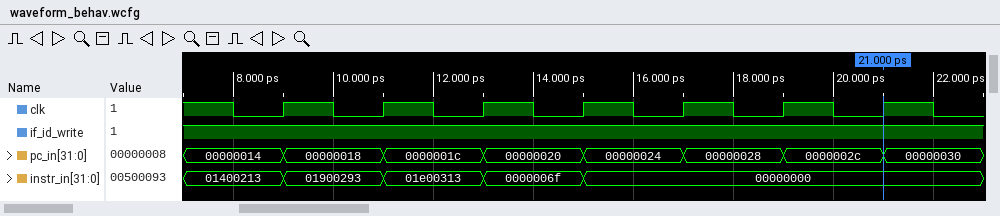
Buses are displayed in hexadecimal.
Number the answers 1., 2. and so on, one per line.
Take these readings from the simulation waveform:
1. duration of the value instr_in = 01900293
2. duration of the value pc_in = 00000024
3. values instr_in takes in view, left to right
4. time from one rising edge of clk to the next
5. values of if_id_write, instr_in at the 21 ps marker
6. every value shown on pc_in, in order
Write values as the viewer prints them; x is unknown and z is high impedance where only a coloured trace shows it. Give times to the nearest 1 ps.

1. 2 ps
2. 2 ps
3. 01400213, 01900293, 01e00313, 0000006f, 00000000
4. 2 ps
5. if_id_write=1, instr_in=00000000
6. 00000014, 00000018, 0000001c, 00000020, 00000024, 00000028, 0000002c, 00000030
